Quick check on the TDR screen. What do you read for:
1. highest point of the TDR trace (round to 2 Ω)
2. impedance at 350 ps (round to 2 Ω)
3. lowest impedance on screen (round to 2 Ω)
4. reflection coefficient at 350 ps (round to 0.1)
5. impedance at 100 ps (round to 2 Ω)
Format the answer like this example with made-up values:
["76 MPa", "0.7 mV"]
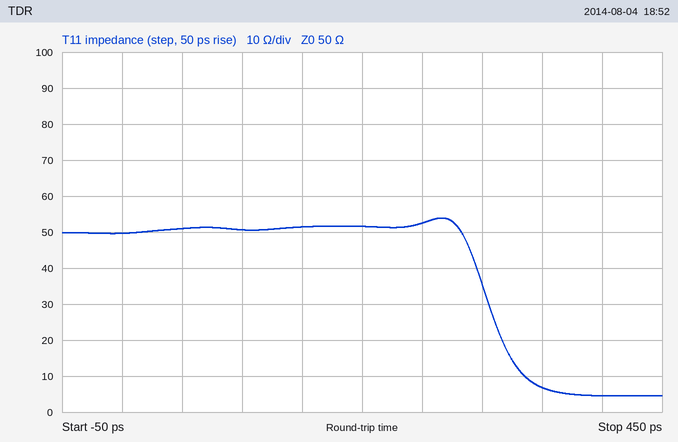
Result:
["54 Ω", "6 Ω", "4 Ω", "-0.8", "50 Ω"]
